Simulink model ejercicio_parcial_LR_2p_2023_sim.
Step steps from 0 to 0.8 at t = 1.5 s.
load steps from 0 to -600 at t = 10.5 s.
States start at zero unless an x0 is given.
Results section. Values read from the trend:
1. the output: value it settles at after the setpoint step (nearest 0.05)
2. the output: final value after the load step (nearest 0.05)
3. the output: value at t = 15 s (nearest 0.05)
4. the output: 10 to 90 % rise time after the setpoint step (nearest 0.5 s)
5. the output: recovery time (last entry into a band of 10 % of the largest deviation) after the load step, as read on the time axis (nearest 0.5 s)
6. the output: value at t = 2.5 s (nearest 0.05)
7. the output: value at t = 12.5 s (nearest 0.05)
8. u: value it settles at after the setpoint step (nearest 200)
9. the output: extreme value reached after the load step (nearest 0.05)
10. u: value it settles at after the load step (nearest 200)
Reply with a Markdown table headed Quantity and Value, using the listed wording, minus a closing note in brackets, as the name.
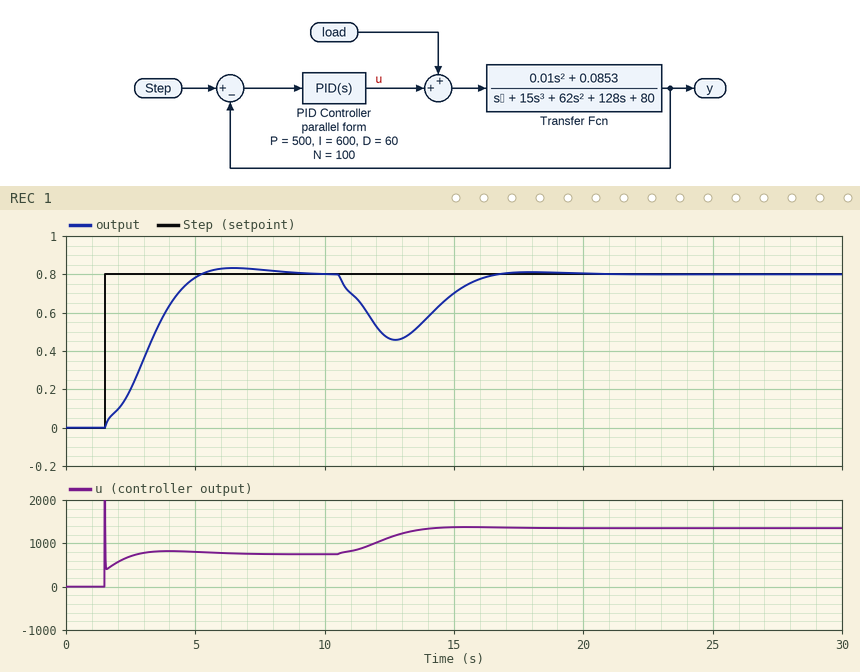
| Quantity | Value |
|---|---|
| the output: value it settles at after the setpoint step | 0.80 |
| the output: final value after the load step | 0.80 |
| the output: value at t = 15 s | 0.70 |
| the output: 10 to 90 % rise time after the setpoint step | 2.5 s |
| the output: recovery time (last entry into a band of 10 % of the largest deviation) after the load step, as read on the time axis | 16.0 s |
| the output: value at t = 2.5 s | 0.20 |
| the output: value at t = 12.5 s | 0.45 |
| u: value it settles at after the setpoint step | 800 |
| the output: extreme value reached after the load step | 0.45 |
| u: value it settles at after the load step | 1400 |
